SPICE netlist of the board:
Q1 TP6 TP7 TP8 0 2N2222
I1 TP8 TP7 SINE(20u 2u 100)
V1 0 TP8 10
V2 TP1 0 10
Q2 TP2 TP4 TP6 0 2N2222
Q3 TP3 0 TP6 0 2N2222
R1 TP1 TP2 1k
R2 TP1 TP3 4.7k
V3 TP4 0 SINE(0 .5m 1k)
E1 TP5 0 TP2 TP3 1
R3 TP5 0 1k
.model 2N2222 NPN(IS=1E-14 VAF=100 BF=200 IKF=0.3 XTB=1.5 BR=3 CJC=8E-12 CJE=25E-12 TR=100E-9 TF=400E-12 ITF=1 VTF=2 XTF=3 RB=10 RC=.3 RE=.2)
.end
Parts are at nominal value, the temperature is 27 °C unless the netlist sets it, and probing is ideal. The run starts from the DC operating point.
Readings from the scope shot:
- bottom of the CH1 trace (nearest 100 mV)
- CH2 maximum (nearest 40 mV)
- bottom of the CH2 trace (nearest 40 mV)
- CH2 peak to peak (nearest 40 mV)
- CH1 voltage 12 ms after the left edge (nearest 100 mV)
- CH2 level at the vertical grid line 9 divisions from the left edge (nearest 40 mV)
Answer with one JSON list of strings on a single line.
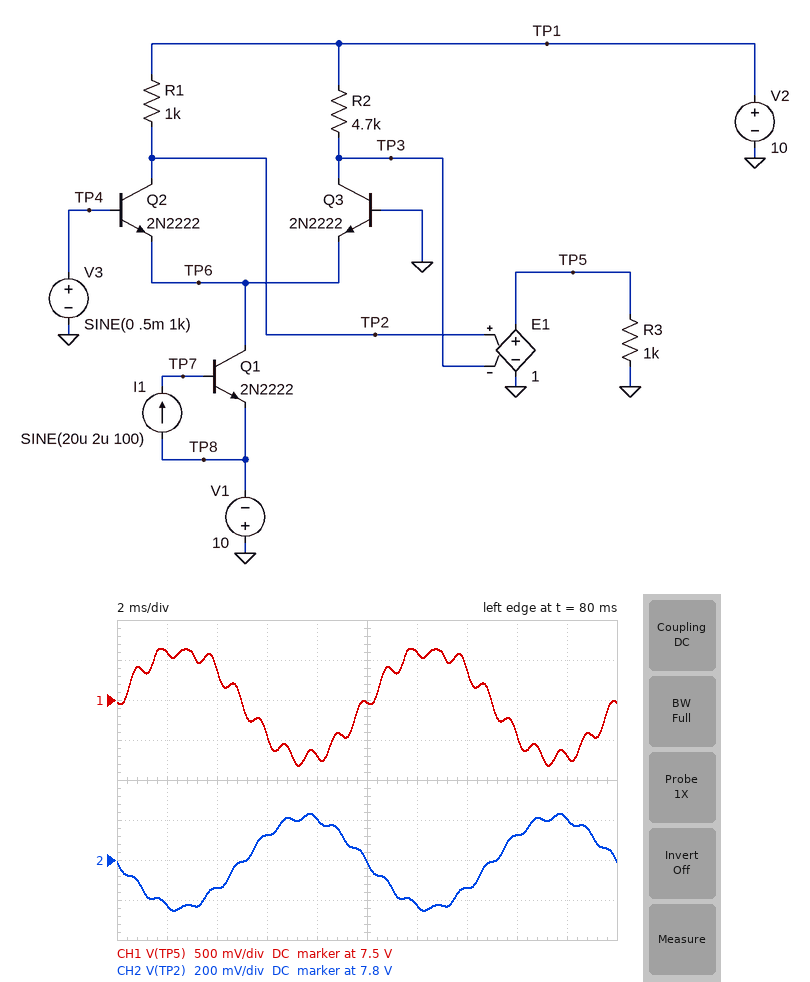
["6.7 V", "8.04 V", "7.56 V", "480 mV", "8.1 V", "8.00 V"]
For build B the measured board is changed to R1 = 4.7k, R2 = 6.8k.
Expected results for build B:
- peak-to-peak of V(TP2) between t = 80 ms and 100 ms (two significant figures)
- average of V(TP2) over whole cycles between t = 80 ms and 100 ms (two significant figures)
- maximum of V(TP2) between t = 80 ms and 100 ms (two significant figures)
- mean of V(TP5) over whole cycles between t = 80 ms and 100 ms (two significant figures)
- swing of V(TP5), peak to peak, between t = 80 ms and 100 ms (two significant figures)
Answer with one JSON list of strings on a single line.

["540 mV", "-550 mV", "-120 mV", "100 mV", "510 mV"]
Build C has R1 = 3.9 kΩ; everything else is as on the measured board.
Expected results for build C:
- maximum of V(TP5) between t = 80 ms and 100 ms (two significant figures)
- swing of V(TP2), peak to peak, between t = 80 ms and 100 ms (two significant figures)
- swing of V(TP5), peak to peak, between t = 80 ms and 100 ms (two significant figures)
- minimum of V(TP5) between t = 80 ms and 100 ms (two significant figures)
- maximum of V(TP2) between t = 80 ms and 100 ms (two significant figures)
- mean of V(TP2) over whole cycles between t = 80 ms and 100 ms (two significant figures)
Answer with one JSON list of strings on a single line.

["1.8 V", "1.9 V", "620 mV", "1.2 V", "2.5 V", "1.6 V"]
